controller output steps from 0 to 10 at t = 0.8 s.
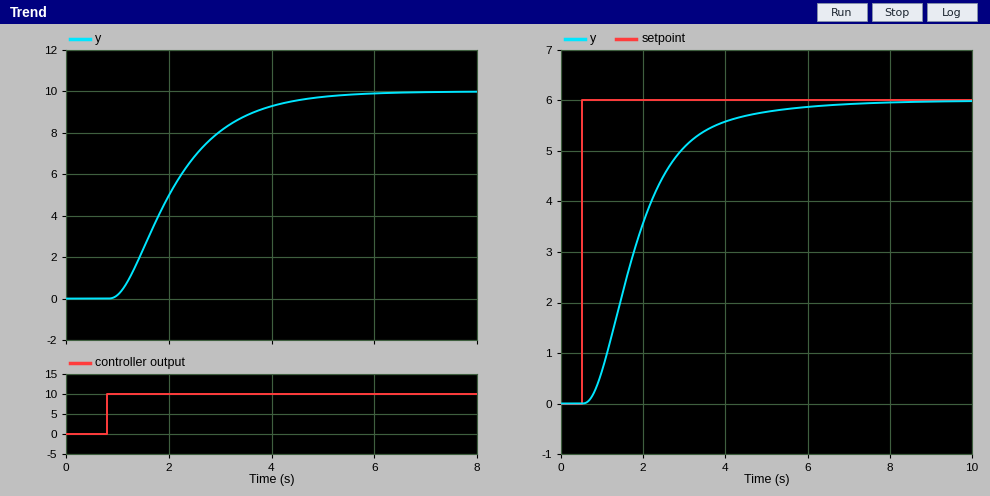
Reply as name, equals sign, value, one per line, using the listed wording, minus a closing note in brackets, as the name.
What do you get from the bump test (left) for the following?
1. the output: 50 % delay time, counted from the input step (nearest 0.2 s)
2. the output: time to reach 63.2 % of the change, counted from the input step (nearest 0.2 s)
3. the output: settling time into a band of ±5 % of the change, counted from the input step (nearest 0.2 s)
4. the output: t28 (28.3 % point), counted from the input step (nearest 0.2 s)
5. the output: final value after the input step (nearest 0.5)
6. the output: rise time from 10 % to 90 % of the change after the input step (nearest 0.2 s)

the output: 50 % delay time, counted from the input step = 1.2 s
the output: time to reach 63.2 % of the change, counted from the input step = 1.6 s
the output: settling time into a band of ±5 % of the change, counted from the input step = 3.6 s
the output: t28 (28.3 % point), counted from the input step = 0.8 s
the output: final value after the input step = 10.0
the output: rise time from 10 % to 90 % of the change after the input step = 2.4 s
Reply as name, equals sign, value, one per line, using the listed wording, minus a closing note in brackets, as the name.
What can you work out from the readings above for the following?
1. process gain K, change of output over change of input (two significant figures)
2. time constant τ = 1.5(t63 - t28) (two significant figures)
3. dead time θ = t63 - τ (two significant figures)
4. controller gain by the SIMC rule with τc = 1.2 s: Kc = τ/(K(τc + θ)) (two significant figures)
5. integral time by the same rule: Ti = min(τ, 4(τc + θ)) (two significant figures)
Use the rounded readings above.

process gain K, change of output over change of input = 1.0
time constant τ = 1.5(t63 - t28) = 1.2 s
dead time θ = t63 - τ = 0.40 s
controller gain by the SIMC rule with τc = 1.2 s: Kc = τ/(K(τc + θ)) = 0.75
integral time by the same rule: Ti = min(τ, 4(τc + θ)) = 1.2 s
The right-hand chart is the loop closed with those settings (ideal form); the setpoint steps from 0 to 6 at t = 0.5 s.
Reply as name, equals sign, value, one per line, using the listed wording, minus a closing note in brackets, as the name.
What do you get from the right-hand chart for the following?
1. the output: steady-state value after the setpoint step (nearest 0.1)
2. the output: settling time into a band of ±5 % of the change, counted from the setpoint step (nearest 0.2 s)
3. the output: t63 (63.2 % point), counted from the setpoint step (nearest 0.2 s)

the output: steady-state value after the setpoint step = 6.0
the output: settling time into a band of ±5 % of the change, counted from the setpoint step = 4.0 s
the output: t63 (63.2 % point), counted from the setpoint step = 1.6 s
